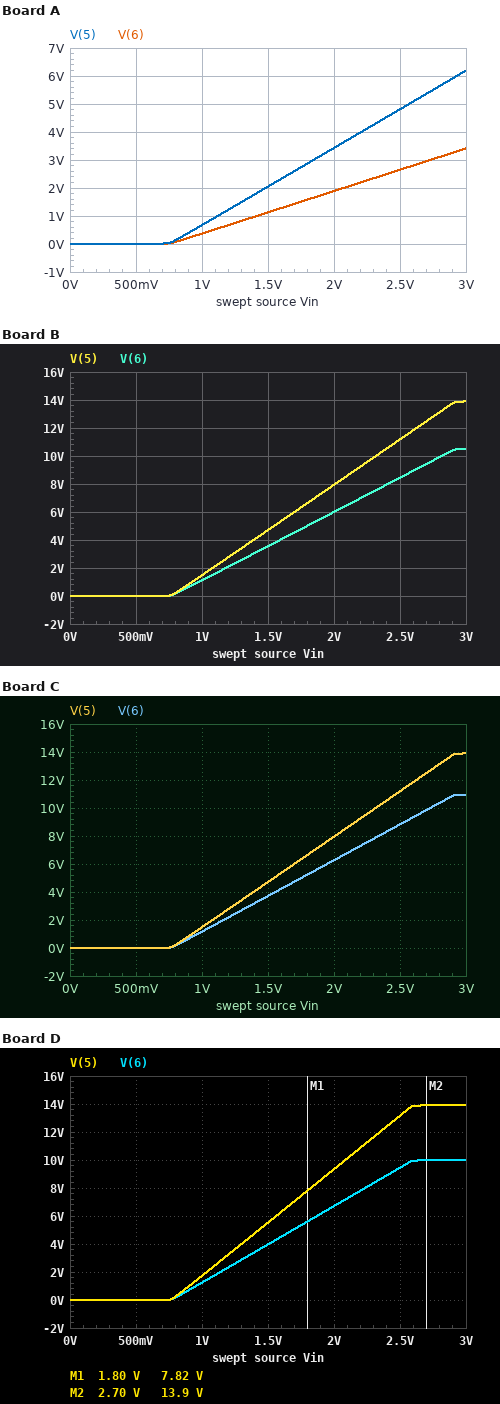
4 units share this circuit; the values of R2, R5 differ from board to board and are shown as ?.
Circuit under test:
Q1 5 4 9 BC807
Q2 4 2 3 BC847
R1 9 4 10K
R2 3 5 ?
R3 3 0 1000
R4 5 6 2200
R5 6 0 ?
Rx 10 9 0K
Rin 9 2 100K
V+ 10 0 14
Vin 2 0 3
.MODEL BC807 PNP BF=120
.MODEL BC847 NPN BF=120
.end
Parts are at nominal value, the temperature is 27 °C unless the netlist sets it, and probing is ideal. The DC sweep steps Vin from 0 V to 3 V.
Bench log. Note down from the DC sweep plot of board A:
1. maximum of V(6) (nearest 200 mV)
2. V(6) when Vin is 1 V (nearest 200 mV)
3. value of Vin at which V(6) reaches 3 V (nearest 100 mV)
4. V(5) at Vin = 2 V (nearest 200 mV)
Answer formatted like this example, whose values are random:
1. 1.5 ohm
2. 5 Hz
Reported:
1. 3.4 V
2. 400 mV
3. 2.7 V
4. 3.4 V
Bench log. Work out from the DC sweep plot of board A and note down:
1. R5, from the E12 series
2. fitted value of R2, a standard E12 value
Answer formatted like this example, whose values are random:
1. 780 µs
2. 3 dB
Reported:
1. 2.7 kΩ
2. 1.8 kΩ
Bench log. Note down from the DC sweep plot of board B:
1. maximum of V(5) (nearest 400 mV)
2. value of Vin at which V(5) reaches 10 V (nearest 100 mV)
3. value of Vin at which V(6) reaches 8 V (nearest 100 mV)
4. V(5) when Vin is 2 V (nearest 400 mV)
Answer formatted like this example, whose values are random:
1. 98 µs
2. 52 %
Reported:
1. 14.0 V
2. 2.3 V
3. 2.4 V
4. 8.0 V
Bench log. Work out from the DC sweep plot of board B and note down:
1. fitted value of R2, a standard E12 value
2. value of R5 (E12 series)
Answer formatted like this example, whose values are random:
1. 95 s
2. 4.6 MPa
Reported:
1. 5.6 kΩ
2. 6.8 kΩ
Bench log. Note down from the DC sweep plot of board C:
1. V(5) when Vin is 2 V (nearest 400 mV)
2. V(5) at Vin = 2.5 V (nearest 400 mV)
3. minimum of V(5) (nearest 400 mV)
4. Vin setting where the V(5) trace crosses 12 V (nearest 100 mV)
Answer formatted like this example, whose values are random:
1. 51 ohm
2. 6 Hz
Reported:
1. 8.0 V
2. 11.2 V
3. 0 V
4. 2.6 V
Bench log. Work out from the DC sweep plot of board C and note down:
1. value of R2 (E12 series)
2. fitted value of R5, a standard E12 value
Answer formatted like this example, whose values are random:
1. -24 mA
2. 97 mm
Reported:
1. 5.6 kΩ
2. 8.2 kΩ
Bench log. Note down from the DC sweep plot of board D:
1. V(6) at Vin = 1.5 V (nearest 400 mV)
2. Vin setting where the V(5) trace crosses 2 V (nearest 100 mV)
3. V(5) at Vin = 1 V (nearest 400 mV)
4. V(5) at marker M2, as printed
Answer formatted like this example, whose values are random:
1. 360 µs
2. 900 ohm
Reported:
1. 4.0 V
2. 1.0 V
3. 1.6 V
4. 13.9 V
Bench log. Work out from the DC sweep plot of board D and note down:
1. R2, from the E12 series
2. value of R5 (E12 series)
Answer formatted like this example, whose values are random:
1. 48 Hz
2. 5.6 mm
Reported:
1. 6.8 kΩ
2. 5.6 kΩ
